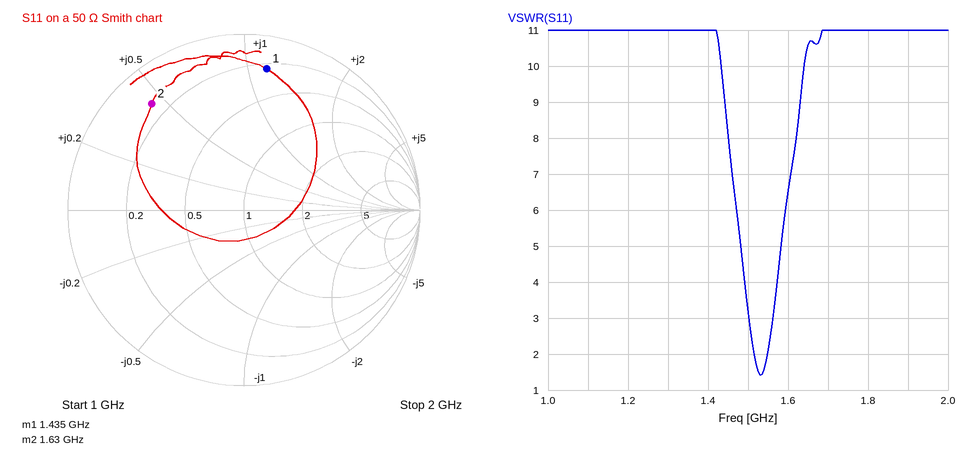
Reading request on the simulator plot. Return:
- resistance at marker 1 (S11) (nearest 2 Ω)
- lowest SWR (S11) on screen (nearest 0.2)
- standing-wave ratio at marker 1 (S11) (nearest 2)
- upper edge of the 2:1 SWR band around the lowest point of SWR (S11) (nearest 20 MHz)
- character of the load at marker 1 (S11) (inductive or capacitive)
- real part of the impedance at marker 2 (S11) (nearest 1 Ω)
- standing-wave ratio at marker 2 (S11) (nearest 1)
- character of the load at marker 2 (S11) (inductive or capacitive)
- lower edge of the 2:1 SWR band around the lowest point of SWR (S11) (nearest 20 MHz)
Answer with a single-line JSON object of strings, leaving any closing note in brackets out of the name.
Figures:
{"resistance at marker 1 (S11)": "12 Ω", "lowest SWR (S11) on screen": "1.4", "standing-wave ratio at marker 1 (S11)": "10", "upper edge of the 2:1 SWR band around the lowest point of SWR (S11)": "1.54 GHz", "character of the load at marker 1 (S11)": "inductive", "real part of the impedance at marker 2 (S11)": "7 Ω", "standing-wave ratio at marker 2 (S11)": "9", "character of the load at marker 2 (S11)": "inductive", "lower edge of the 2:1 SWR band around the lowest point of SWR (S11)": "1.52 GHz"}
